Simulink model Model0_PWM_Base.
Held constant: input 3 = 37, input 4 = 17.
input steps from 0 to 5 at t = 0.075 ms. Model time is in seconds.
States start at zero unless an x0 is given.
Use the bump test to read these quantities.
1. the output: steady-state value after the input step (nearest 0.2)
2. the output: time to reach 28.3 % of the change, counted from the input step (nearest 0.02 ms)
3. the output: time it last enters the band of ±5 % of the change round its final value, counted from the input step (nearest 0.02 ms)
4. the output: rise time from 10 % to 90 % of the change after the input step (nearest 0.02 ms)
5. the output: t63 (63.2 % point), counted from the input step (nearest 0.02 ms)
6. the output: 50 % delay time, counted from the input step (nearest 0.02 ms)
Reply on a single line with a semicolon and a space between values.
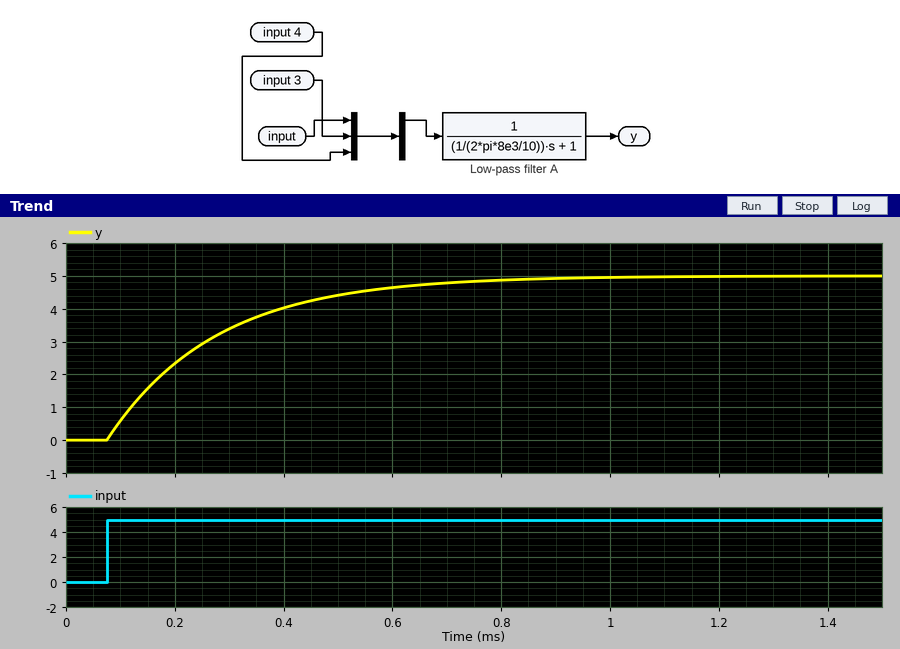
5.0; 0.06 ms; 0.60 ms; 0.44 ms; 0.20 ms; 0.14 ms
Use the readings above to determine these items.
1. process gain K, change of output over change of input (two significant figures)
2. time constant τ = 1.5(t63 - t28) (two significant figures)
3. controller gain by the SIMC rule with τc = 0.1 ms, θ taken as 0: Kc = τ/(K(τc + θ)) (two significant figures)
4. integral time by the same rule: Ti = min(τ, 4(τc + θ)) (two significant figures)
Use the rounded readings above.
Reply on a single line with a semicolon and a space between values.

1.0; 0.21 ms; 2.1; 0.21 ms
